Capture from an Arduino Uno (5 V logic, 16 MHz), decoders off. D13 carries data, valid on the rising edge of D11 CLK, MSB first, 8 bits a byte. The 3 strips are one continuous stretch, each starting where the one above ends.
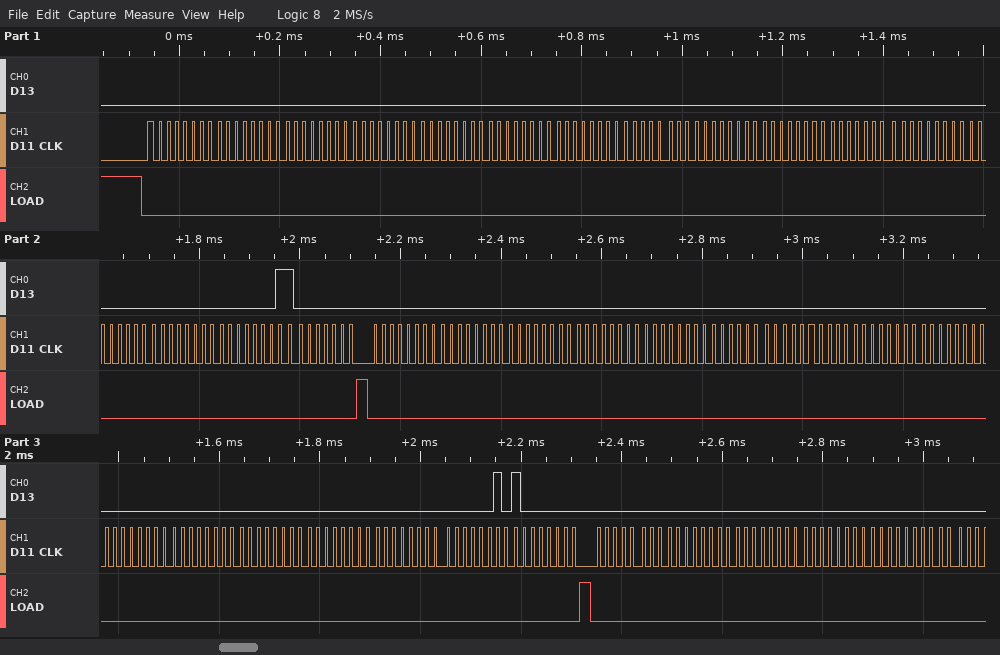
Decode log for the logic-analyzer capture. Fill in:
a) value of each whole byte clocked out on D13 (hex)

0x00 0x00 0x00 0x00 0x00 0x00 0x00 0x00 0x00 0x00 0x00 0x00 0x00 0x00 0x01 0x80 0x00 0x00 0x00 0x00 0x00 0x00 0x00 0x00 0x00 0x00 0x00 0x00 0x00 0x00 0x02 0x80 0x00 0x00 0x00 0x00 0x00
